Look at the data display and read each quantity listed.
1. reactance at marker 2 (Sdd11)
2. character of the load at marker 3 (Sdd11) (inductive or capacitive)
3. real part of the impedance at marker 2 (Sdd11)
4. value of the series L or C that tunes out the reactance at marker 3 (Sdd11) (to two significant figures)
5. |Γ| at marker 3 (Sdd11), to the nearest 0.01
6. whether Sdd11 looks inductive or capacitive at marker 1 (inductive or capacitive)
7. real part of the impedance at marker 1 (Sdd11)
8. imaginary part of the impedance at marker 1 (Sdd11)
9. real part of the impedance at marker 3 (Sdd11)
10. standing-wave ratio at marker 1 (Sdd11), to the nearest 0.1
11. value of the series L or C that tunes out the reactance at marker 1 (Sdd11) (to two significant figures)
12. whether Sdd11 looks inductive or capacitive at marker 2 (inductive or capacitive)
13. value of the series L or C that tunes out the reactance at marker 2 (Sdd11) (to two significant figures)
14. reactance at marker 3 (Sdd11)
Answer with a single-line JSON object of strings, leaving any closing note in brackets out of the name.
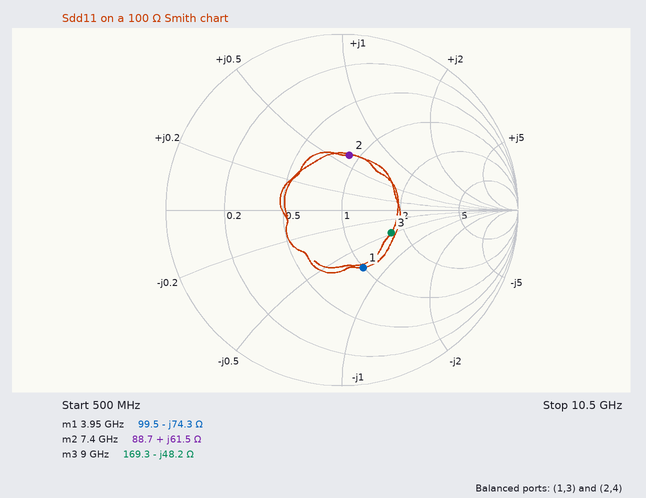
{"reactance at marker 2": "+61.5 Ω", "character of the load at marker 3 (Sdd11)": "capacitive", "real part of the impedance at marker 2": "88.7 Ω", "value of the series L or C that tunes out the reactance at marker 3 (Sdd11)": "850 pH", "|Γ| at marker 3 (Sdd11), to the nearest 0.01": "0.31", "whether Sdd11 looks inductive or capacitive at marker 1": "capacitive", "real part of the impedance at marker 1": "99.5 Ω", "imaginary part of the impedance at marker 1": "-74.3 Ω", "real part of the impedance at marker 3": "169.3 Ω", "standing-wave ratio at marker 1 (Sdd11), to the nearest 0.1": "2.1", "value of the series L or C that tunes out the reactance at marker 1 (Sdd11)": "3.0 nH", "whether Sdd11 looks inductive or capacitive at marker 2": "inductive", "value of the series L or C that tunes out the reactance at marker 2 (Sdd11)": "350 fF", "reactance at marker 3": "-48.2 Ω"}
